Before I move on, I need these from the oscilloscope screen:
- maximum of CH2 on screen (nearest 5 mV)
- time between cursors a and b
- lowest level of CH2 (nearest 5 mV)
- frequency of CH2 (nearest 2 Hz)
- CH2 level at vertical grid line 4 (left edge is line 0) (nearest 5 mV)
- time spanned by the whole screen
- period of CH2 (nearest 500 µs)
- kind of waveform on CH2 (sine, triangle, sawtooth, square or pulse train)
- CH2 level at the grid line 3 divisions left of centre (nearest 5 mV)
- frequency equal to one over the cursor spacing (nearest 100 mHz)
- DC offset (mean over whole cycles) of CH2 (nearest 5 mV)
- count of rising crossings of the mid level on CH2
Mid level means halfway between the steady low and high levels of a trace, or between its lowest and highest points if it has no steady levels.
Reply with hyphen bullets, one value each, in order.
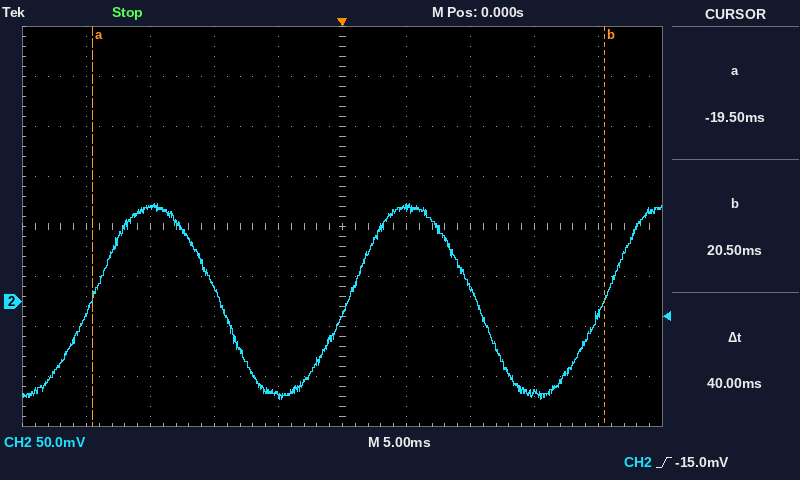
- 100 mV
- 40 ms
- -100 mV
- 50 Hz
- -95 mV
- 50 ms
- 20.0 ms
- sine
- 95 mV
- 25.0 Hz
- 0 mV
- 3
